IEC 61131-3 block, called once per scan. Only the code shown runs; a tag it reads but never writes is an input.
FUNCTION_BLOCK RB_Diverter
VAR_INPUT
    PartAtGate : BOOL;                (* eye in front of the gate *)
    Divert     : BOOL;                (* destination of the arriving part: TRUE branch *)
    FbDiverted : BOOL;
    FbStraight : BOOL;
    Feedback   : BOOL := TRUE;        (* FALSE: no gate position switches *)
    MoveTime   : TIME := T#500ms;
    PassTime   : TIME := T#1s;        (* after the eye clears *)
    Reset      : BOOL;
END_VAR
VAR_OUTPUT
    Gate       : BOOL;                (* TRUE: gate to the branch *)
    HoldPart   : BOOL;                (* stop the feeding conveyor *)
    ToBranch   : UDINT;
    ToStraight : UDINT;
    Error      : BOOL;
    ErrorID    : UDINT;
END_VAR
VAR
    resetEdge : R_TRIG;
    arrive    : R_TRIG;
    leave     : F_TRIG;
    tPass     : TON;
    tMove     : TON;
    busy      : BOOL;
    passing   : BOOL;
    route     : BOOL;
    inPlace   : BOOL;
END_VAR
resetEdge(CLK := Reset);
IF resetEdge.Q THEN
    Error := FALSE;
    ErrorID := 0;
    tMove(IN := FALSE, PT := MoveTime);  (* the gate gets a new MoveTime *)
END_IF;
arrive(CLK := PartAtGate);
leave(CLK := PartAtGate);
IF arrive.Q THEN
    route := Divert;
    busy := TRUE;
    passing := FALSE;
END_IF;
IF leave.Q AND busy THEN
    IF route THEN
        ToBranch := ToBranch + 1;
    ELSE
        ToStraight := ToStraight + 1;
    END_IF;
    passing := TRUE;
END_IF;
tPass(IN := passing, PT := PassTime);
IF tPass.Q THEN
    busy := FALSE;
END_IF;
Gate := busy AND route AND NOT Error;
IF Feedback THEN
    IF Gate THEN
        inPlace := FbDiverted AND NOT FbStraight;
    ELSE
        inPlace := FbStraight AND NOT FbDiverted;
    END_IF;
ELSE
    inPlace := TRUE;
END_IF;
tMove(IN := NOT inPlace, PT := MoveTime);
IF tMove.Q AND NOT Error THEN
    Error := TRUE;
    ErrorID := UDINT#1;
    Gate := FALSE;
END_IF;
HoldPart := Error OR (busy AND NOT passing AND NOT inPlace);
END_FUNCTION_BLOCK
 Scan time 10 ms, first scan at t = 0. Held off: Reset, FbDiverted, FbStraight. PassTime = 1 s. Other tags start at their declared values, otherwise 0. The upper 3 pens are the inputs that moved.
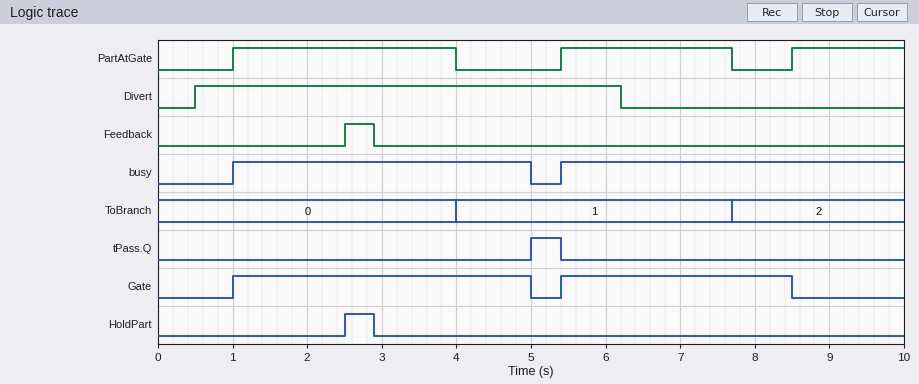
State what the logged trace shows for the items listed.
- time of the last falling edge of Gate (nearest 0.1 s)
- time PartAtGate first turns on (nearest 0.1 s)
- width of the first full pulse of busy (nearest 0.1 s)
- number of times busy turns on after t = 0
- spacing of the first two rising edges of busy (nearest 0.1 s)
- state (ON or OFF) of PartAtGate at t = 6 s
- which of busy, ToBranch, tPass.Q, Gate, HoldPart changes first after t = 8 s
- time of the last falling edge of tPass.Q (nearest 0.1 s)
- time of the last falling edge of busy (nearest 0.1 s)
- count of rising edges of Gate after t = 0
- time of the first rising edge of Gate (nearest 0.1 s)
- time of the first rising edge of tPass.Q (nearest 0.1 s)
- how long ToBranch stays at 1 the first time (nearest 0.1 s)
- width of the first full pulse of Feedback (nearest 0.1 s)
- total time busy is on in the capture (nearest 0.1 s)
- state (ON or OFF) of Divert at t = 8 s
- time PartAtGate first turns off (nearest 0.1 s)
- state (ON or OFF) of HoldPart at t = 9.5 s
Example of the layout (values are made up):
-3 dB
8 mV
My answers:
8.5 s
1.0 s
4.0 s
2
4.4 s
ON
Gate
5.4 s
5.0 s
2
1.0 s
5.0 s
3.7 s
0.4 s
8.6 s
OFF
4.0 s
OFF
